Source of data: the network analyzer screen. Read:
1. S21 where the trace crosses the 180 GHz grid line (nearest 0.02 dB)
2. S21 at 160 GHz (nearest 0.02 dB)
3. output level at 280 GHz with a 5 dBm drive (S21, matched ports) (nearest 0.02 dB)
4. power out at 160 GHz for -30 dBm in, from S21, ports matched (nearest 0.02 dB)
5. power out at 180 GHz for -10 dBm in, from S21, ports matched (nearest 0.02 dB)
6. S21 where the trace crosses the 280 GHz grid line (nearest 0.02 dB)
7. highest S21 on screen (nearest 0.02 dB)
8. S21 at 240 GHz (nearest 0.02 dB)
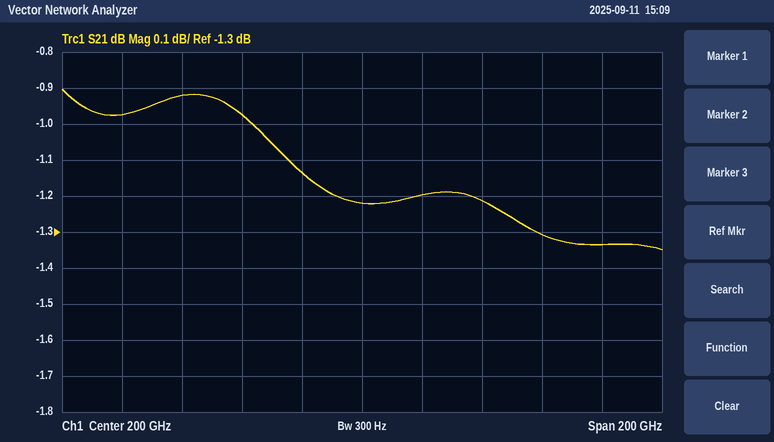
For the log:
-1.14 dB
-0.98 dB
3.66 dBm
-30.98 dBm
-11.14 dBm
-1.34 dB
-0.90 dB
-1.22 dB
